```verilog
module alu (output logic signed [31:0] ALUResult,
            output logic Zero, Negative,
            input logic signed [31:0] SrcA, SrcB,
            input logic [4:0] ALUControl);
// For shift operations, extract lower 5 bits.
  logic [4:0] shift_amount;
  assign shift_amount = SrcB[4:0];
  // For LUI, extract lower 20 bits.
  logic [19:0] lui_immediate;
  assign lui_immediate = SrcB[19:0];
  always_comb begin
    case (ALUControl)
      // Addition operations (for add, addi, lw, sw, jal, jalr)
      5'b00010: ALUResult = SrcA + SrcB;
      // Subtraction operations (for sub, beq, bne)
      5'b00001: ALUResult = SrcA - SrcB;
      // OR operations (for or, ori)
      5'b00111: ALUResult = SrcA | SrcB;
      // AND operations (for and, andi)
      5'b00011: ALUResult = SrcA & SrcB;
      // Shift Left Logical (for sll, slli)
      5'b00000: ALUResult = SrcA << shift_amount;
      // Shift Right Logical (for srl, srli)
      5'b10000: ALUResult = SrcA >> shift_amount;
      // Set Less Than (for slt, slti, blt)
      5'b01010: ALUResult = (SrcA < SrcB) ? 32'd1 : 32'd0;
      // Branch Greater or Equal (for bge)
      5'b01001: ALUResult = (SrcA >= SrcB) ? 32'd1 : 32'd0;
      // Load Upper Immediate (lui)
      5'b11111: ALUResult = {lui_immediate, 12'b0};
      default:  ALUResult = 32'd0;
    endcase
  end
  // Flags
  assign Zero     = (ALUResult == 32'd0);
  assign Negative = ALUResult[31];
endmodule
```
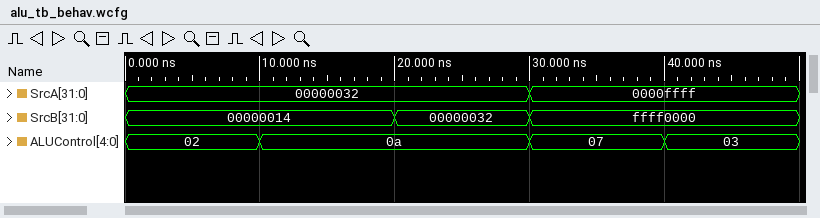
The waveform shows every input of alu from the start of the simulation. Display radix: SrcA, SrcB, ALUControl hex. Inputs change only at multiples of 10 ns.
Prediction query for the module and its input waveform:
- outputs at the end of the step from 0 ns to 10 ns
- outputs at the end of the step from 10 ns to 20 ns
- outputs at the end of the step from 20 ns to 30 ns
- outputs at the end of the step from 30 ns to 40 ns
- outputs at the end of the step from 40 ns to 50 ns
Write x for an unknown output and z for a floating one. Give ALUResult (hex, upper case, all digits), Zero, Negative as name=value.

ALUResult=00000046, Zero=0, Negative=0
ALUResult=00000000, Zero=1, Negative=0
ALUResult=00000000, Zero=1, Negative=0
ALUResult=FFFFFFFF, Zero=0, Negative=1
ALUResult=00000000, Zero=1, Negative=0
